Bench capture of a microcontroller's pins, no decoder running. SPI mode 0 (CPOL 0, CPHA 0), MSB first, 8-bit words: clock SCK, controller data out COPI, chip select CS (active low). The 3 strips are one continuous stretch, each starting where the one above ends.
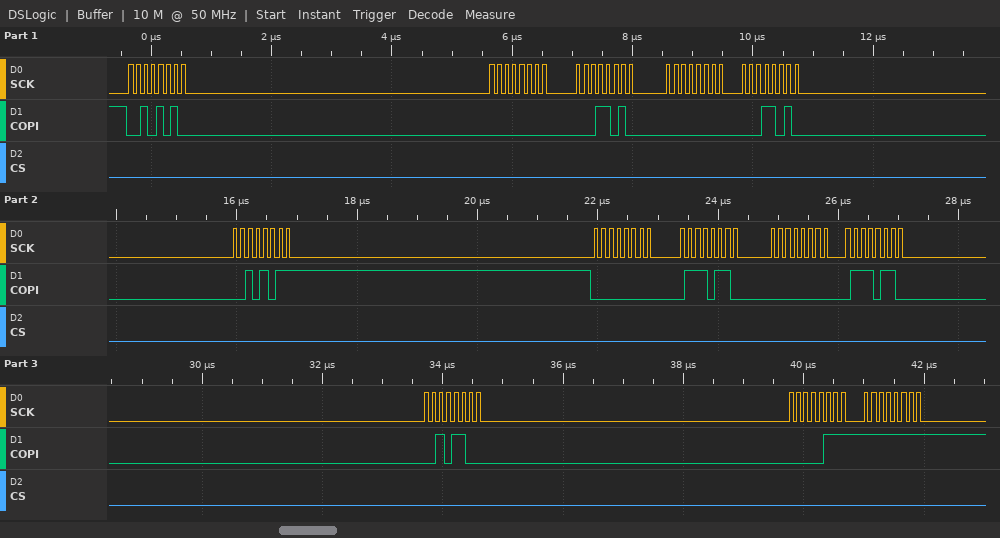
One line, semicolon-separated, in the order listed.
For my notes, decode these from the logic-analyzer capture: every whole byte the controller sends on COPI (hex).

2A 00 1A 00 1A 2B 00 76 00 76 2C 07 FF
